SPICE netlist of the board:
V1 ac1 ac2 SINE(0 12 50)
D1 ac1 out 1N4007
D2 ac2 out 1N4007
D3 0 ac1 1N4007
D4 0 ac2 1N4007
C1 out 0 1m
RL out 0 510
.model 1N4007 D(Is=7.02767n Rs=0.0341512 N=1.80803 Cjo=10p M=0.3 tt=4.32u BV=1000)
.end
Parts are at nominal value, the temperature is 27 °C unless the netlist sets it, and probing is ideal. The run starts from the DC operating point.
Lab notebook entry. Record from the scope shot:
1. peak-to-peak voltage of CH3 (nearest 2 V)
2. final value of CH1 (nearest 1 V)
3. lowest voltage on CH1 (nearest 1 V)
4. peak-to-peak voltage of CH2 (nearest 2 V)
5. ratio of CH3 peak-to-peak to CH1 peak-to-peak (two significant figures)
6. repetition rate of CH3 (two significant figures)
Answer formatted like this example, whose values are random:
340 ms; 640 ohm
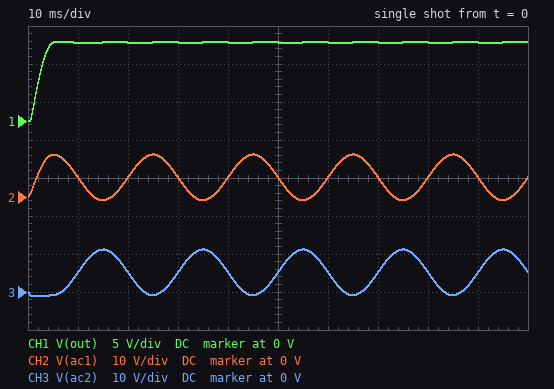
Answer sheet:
12 V; 10 V; 0 V; 12 V; 1.2; 50 Hz
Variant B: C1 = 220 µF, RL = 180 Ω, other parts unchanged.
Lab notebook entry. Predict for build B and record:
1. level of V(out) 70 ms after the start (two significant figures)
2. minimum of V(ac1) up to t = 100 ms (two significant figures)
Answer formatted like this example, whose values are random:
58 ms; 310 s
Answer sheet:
9.3 V; -850 mV
